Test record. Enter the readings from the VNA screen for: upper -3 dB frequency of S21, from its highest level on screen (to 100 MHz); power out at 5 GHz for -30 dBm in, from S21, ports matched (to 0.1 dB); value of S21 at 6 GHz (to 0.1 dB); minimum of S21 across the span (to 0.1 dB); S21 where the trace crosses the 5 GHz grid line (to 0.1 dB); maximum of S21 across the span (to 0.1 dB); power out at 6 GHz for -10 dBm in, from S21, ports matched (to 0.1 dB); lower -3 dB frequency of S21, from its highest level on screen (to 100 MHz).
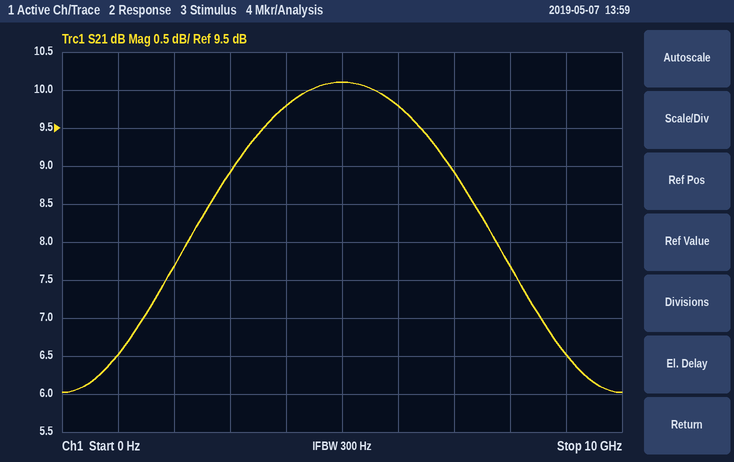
8.5 GHz
-19.9 dBm
9.8 dB
6.0 dB
10.1 dB
10.1 dB
-0.2 dBm
1.5 GHz
